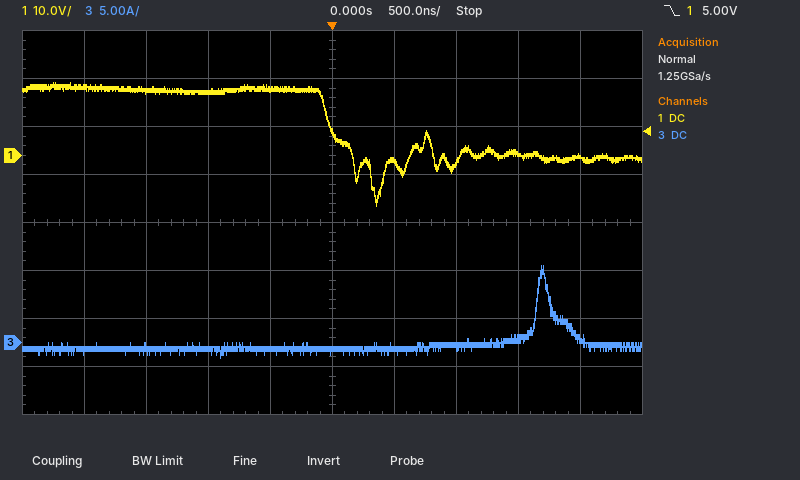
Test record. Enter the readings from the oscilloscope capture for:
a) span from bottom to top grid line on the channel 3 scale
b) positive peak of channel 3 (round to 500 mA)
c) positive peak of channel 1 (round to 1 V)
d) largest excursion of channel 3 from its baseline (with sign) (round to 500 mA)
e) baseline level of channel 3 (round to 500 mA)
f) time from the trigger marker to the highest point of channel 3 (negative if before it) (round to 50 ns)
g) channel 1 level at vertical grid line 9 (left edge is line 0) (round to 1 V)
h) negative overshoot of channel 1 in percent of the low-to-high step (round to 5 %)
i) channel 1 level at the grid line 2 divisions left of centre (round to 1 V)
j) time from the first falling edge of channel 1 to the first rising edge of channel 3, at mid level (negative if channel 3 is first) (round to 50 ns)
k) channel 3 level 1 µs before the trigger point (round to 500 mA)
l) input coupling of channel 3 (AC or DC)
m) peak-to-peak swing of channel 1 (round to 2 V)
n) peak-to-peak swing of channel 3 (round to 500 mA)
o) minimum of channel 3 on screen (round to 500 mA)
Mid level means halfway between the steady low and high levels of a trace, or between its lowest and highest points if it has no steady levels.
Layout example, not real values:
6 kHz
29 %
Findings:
40 A
8.0 A
15 V
+8.5 A
-500 mA
+1.70 µs
0 V
70 %
13 V
+1.65 µs
-500 mA
DC
26 V
9.5 A
-1.5 A
